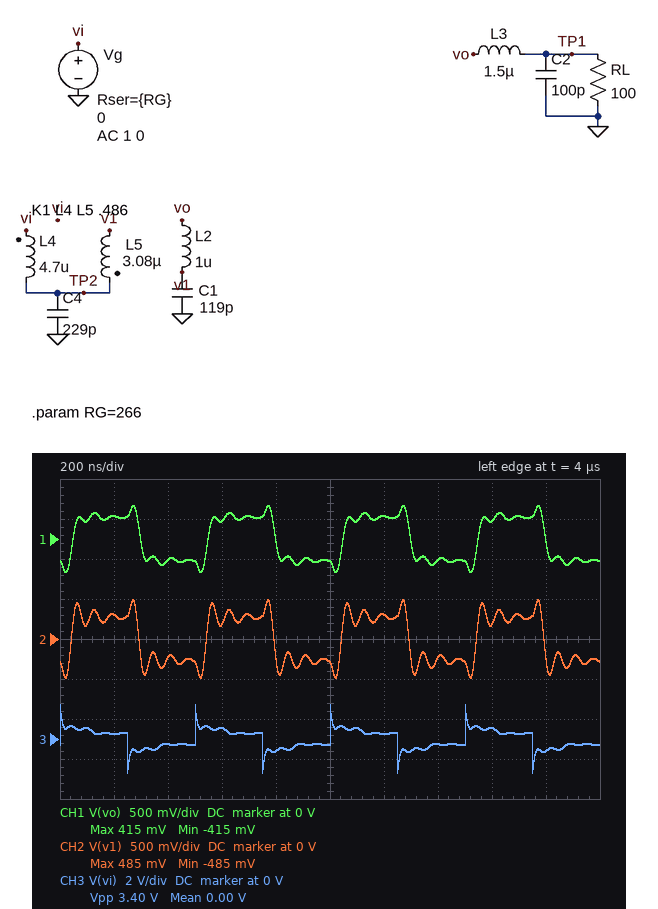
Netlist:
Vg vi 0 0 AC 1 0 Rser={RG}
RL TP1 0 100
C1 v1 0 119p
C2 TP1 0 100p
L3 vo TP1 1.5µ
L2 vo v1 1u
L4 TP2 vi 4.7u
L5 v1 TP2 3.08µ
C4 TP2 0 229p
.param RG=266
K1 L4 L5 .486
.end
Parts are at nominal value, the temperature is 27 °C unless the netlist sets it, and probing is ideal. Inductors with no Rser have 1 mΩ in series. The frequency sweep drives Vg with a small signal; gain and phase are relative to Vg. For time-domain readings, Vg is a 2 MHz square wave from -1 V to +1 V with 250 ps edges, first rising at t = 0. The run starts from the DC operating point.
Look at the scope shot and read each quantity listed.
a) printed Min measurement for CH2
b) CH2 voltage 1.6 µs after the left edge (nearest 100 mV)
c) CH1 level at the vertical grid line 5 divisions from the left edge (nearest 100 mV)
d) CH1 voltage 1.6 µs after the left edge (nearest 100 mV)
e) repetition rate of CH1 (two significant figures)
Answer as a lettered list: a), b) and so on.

a) -485 mV
b) 200 mV
c) -300 mV
d) 200 mV
e) 2.0 MHz
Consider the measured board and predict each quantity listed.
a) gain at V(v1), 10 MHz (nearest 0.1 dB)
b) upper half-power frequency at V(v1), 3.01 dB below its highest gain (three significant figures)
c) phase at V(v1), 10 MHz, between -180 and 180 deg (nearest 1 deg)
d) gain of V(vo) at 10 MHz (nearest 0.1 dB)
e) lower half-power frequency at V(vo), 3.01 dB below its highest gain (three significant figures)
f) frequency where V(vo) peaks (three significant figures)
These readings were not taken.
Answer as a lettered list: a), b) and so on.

a) -7.6 dB
b) 16.8 MHz
c) -145 deg
d) -11.3 dB
e) 12.2 MHz
f) 15.0 MHz
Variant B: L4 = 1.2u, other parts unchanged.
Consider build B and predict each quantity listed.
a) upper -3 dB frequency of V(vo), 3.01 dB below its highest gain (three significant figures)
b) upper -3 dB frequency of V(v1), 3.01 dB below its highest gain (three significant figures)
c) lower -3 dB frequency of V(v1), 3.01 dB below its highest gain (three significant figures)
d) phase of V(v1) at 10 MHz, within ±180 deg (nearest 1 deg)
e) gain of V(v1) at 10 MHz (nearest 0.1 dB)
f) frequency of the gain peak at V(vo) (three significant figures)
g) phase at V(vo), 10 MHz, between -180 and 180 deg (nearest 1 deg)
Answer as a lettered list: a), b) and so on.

a) 15.7 MHz
b) 15.8 MHz
c) 11.7 MHz
d) -118 deg
e) -8.3 dB
f) 13.9 MHz
g) -141 deg
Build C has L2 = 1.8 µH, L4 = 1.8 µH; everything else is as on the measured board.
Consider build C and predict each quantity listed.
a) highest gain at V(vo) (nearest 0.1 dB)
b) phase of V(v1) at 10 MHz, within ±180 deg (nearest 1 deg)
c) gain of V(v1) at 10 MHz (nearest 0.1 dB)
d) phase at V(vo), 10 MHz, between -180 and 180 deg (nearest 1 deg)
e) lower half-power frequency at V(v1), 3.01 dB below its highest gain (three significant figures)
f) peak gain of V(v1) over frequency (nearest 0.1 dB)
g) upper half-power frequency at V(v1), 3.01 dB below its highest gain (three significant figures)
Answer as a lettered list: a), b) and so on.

a) -9.0 dB
b) -124 deg
c) -5.6 dB
d) -156 deg
e) 10.8 MHz
f) -1.4 dB
g) 14.9 MHz
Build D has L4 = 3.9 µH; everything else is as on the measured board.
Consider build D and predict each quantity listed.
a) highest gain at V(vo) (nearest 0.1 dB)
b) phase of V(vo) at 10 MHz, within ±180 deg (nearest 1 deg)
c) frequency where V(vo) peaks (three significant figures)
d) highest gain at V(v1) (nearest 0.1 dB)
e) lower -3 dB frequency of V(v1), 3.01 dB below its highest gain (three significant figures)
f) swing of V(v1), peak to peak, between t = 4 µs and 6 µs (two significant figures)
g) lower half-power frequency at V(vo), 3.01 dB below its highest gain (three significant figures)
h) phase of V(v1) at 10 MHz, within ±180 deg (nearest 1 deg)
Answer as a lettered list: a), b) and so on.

a) -7.5 dB
b) -163 deg
c) 14.8 MHz
d) -2.3 dB
e) 12.3 MHz
f) 960 mV
g) 11.7 MHz
h) -140 deg
